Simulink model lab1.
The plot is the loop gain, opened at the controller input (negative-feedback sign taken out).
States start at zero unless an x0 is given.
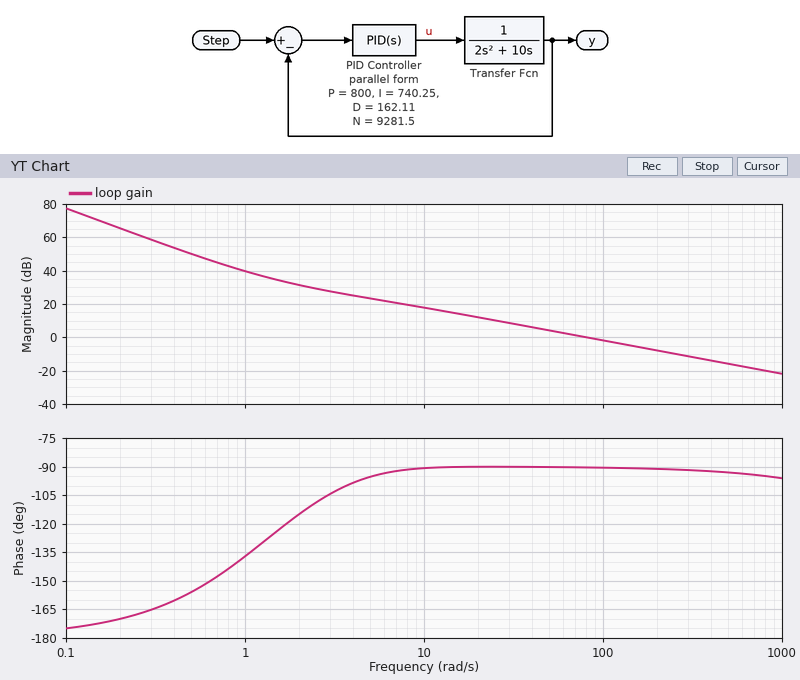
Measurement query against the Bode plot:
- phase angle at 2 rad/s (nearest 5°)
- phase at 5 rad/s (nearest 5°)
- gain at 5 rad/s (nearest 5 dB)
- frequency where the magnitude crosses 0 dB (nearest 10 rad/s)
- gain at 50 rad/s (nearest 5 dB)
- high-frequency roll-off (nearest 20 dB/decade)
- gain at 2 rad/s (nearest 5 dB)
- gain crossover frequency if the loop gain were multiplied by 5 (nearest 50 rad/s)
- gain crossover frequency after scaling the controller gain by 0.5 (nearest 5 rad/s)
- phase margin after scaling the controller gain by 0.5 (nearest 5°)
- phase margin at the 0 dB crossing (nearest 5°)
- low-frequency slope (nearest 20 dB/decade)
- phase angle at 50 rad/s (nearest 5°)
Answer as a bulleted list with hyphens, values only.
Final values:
- -115°
- -95°
- 25 dB
- 80 rad/s
- 5 dB
- -20 dB/decade
- 30 dB
- 400 rad/s
- 40 rad/s
- 90°
- 90°
- -40 dB/decade
- -90°
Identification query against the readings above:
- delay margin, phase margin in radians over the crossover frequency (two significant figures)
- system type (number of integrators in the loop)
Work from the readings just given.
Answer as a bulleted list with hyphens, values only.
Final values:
- 0.020 s
- 2
